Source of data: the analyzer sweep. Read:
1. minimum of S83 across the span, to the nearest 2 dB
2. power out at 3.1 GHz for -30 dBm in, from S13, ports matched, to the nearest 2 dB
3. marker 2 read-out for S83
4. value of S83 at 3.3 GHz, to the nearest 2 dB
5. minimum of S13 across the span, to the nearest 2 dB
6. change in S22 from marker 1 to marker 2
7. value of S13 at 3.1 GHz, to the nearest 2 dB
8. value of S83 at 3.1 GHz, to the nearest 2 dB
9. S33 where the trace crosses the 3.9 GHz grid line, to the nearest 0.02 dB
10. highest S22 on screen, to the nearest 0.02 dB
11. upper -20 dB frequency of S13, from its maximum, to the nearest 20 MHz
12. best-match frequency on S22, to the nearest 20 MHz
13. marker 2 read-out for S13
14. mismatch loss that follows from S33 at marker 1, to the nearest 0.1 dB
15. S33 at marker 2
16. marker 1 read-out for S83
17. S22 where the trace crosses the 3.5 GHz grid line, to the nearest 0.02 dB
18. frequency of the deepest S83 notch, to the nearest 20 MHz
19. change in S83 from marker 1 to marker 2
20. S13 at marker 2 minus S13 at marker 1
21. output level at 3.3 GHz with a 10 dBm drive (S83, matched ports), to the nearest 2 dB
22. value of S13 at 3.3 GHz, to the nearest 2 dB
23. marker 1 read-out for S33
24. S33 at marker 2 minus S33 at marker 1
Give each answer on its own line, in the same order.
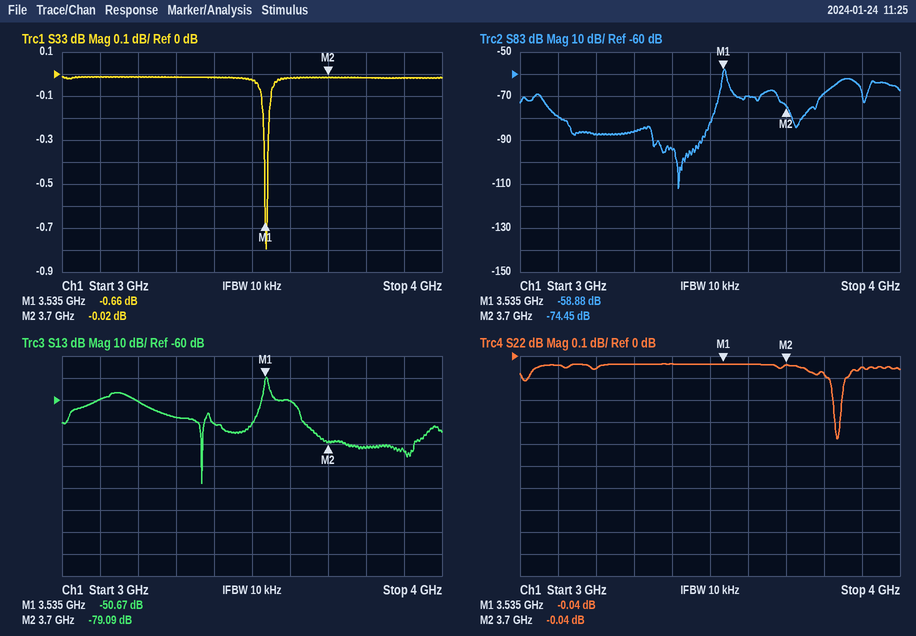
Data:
-112 dB
-90 dBm
-74.45 dB
-86 dB
-98 dB
0.00 dB
-60 dB
-80 dB
-0.02 dB
-0.04 dB
3.64 GHz
3.84 GHz
-79.09 dB
8.5 dB
-0.02 dB
-58.88 dB
-0.04 dB
3.42 GHz
-15.57 dB
-28.42 dB
-76 dBm
-68 dB
-0.66 dB
0.64 dB
